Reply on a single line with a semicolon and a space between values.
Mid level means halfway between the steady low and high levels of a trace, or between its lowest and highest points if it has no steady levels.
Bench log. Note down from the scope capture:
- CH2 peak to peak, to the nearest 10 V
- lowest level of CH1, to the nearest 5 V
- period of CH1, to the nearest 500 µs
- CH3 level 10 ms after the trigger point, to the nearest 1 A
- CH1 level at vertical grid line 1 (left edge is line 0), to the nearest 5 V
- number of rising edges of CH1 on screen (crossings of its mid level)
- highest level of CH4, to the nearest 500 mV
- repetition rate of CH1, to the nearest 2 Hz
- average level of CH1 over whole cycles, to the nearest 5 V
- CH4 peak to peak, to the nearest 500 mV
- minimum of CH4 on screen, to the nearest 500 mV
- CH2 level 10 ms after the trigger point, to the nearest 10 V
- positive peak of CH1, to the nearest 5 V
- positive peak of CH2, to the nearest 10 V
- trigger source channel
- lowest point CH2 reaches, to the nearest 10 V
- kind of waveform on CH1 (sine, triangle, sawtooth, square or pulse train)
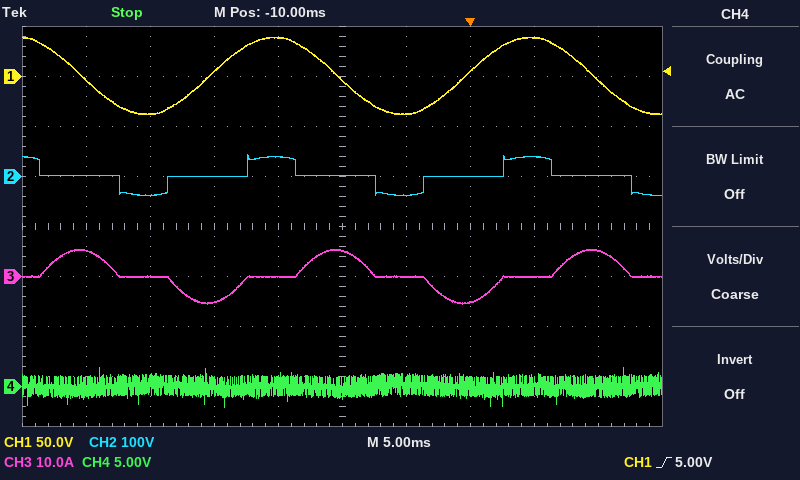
80 V; -40 V; 20.0 ms; 5 A; -5 V; 2; 2.0 V; 50 Hz; 0 V; 4.0 V; -2.0 V; 0 V; 40 V; 40 V; CH1; -40 V; sine
